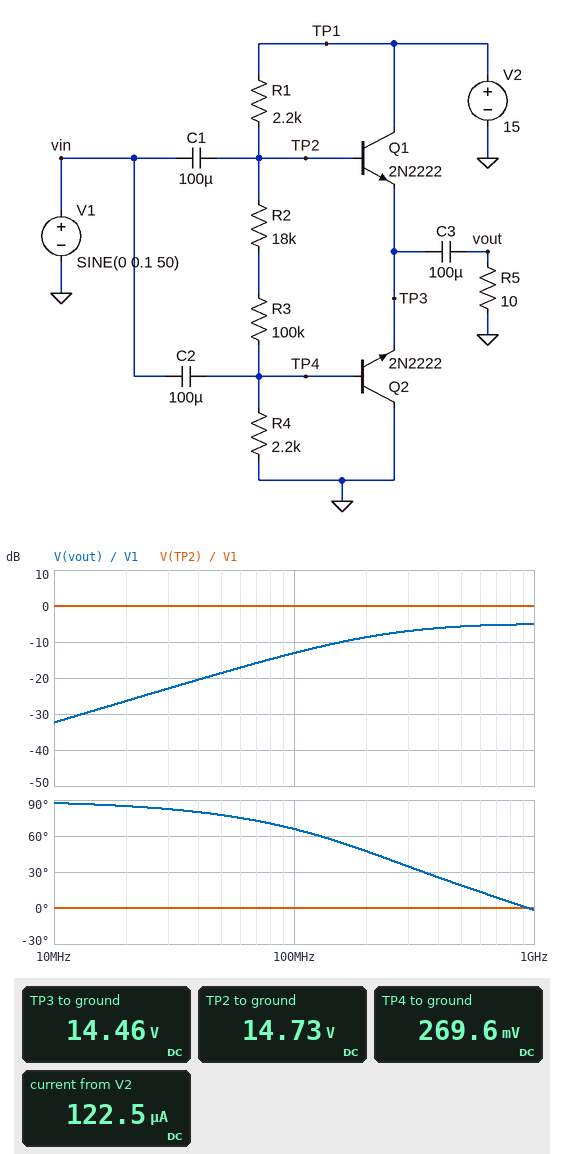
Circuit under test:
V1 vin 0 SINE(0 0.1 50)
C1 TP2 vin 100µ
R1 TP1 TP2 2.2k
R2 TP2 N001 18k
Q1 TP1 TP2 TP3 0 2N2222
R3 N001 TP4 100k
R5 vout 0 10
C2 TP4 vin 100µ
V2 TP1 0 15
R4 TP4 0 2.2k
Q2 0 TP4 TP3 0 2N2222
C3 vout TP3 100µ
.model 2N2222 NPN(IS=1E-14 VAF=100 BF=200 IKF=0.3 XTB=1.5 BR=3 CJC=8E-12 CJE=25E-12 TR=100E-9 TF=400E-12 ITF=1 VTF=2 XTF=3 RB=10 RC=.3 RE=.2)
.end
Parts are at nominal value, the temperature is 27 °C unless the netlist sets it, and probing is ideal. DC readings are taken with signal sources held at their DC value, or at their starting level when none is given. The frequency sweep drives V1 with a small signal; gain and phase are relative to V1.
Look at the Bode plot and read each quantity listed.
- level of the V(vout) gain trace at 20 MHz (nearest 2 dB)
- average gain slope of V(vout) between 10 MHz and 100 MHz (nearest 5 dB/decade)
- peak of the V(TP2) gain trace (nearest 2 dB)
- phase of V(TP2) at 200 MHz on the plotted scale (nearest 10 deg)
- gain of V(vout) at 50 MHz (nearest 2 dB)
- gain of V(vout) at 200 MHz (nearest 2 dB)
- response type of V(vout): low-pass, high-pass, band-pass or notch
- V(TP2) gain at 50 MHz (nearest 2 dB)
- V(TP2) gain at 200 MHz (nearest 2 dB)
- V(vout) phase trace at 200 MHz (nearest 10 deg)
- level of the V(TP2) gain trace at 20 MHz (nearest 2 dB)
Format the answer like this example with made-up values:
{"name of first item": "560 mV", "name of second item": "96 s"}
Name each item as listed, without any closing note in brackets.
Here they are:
{"level of the V(vout) gain trace at 20 MHz": "-26 dB", "average gain slope of V(vout) between 10 MHz and 100 MHz": "20 dB/decade", "peak of the V(TP2) gain trace": "0 dB", "phase of V(TP2) at 200 MHz on the plotted scale": "0 deg", "gain of V(vout) at 50 MHz": "-18 dB", "gain of V(vout) at 200 MHz": "-8 dB", "response type of V(vout): low-pass, high-pass, band-pass or notch": "high-pass", "V(TP2) gain at 50 MHz": "0 dB", "V(TP2) gain at 200 MHz": "0 dB", "V(vout) phase trace at 200 MHz": "50 deg", "level of the V(TP2) gain trace at 20 MHz": "0 dB"}
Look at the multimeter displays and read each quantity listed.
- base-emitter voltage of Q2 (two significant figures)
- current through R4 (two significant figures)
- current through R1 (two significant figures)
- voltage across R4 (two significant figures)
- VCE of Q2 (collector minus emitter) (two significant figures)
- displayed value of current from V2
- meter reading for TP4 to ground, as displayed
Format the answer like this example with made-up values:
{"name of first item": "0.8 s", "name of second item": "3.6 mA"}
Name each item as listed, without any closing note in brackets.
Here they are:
{"base-emitter voltage of Q2": "-14 V", "current through R4": "120 µA", "current through R1": "120 µA", "voltage across R4": "270 mV", "VCE of Q2 (collector minus emitter)": "-14 V", "displayed value of current from V2": "122.5 µA", "meter reading for TP4 to ground, as displayed": "269.6 mV"}
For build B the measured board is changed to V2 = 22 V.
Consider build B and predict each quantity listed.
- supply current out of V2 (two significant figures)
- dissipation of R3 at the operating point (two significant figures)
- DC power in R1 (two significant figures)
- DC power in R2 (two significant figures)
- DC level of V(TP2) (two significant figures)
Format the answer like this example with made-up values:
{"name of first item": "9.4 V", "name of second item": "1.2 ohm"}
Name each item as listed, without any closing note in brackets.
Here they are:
{"supply current out of V2": "180 µA", "dissipation of R3 at the operating point": "3.2 mW", "DC power in R1": "71 µW", "DC power in R2": "580 µW", "DC level of V(TP2)": "22 V"}
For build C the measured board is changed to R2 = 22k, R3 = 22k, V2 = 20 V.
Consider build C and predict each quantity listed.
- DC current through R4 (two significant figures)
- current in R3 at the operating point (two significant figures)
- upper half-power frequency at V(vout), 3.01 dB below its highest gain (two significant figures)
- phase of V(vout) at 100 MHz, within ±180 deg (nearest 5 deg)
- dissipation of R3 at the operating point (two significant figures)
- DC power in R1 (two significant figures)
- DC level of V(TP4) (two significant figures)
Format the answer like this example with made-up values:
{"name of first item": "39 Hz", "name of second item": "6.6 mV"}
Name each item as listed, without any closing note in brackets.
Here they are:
{"DC current through R4": "290 µA", "current in R3 at the operating point": "420 µA", "upper half-power frequency at V(vout), 3.01 dB below its highest gain": "2.4 GHz", "phase of V(vout) at 100 MHz, within ±180 deg": "35 deg", "dissipation of R3 at the operating point": "3.9 mW", "DC power in R1": "390 µW", "DC level of V(TP4)": "630 mV"}
